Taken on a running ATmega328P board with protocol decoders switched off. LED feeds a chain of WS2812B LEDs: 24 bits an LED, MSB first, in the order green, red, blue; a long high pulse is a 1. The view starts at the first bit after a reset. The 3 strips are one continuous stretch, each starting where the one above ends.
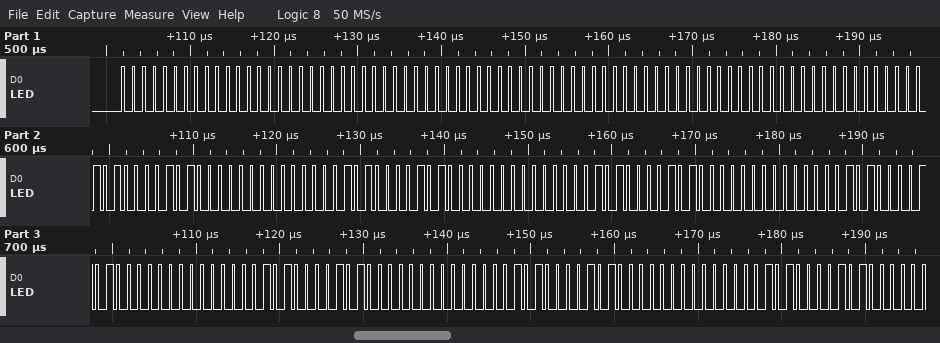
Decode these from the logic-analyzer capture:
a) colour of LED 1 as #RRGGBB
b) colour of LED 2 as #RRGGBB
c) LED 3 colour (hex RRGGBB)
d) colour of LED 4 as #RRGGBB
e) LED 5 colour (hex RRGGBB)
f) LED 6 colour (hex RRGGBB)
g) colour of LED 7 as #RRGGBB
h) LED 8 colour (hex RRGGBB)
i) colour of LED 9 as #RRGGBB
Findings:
#000000
#000000
#000000
#0A0500
#0A0500
#0A0500
#0A0500
#0A0500
#0A0500
